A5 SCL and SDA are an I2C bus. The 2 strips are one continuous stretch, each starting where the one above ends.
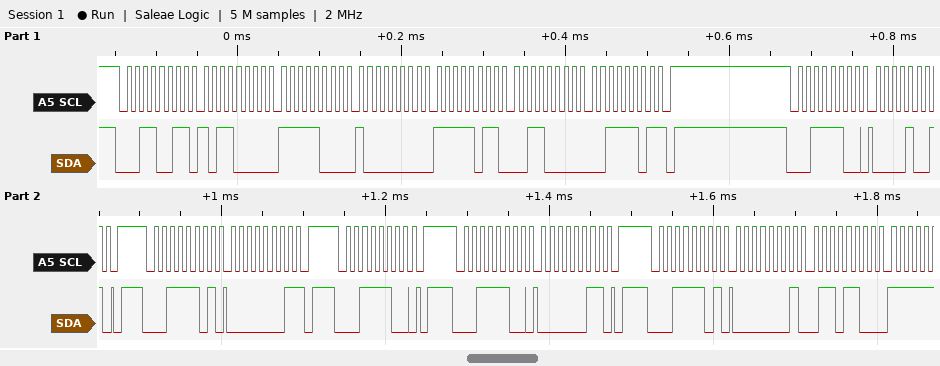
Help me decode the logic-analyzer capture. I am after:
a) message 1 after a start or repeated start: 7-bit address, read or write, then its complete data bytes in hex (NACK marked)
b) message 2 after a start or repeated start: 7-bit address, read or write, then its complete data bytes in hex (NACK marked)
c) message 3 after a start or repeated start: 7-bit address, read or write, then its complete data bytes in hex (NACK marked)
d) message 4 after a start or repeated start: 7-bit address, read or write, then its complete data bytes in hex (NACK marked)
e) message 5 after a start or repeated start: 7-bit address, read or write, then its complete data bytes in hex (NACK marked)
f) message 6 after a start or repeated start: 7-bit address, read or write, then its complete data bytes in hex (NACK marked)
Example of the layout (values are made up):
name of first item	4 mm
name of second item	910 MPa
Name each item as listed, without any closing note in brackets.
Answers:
message 1 after a start or repeated start: 7-bit address, read or write, then its complete data bytes in hex	0x19 read: B0 F8 80 FB 30 3D NACK
message 2 after a start or repeated start: 7-bit address, read or write, then its complete data bytes in hex	0x1E write: 09
message 3 after a start or repeated start: 7-bit address, read or write, then its complete data bytes in hex	0x1E read: 01 NACK
message 4 after a start or repeated start: 7-bit address, read or write, then its complete data bytes in hex	0x1E write
message 5 after a start or repeated start: 7-bit address, read or write, then its complete data bytes in hex	0x1E write: 03
message 6 after a start or repeated start: 7-bit address, read or write, then its complete data bytes in hex	0x1E read: 01 6C
